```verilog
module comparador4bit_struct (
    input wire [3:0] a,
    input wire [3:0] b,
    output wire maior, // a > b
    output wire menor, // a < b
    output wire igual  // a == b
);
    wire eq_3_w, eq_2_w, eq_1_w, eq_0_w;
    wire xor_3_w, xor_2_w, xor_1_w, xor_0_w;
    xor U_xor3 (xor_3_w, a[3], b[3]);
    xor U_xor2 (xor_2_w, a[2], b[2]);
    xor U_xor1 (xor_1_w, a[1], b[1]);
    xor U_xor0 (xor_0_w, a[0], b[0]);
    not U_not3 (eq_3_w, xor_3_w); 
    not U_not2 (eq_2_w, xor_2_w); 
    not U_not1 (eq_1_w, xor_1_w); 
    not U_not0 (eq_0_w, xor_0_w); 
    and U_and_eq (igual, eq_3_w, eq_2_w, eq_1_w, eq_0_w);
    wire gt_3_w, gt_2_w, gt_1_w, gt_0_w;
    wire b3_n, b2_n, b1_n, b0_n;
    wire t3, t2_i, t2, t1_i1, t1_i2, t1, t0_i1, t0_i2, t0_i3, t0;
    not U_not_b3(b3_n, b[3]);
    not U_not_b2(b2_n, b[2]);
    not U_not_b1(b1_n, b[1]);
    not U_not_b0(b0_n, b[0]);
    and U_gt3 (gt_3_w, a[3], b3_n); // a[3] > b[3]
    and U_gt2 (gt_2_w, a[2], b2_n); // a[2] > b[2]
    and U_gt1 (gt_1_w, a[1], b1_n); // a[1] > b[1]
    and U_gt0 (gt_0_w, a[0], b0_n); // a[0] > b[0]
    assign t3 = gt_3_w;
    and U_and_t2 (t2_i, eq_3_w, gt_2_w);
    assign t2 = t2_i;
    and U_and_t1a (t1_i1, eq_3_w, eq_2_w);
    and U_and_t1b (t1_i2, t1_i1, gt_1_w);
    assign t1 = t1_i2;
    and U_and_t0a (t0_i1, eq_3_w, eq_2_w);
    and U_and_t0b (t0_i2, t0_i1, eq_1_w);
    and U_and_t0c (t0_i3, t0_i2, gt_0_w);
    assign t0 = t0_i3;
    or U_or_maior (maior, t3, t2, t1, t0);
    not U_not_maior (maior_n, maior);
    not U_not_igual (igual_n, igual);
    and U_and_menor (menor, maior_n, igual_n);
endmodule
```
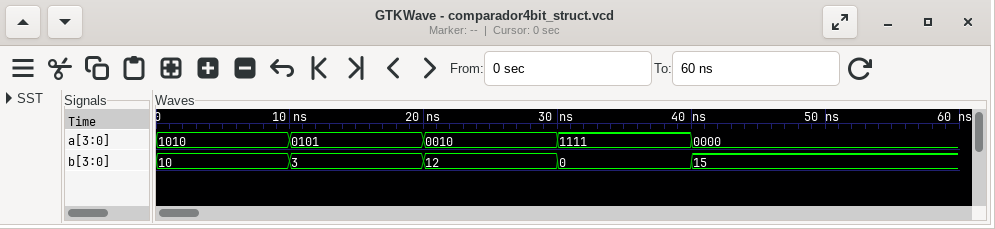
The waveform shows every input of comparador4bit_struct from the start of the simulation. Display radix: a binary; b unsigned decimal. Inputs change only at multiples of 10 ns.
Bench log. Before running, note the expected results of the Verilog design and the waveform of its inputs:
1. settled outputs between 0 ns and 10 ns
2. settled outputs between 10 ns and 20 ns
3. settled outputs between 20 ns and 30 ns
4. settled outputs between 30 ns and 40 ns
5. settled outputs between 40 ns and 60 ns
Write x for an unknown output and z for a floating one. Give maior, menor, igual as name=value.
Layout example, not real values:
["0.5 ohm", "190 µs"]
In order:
["maior=0, menor=0, igual=1", "maior=1, menor=0, igual=0", "maior=0, menor=1, igual=0", "maior=1, menor=0, igual=0", "maior=0, menor=1, igual=0"]
